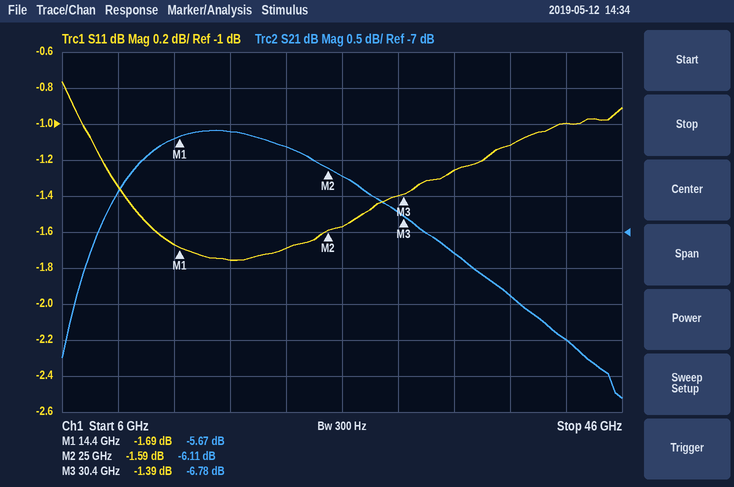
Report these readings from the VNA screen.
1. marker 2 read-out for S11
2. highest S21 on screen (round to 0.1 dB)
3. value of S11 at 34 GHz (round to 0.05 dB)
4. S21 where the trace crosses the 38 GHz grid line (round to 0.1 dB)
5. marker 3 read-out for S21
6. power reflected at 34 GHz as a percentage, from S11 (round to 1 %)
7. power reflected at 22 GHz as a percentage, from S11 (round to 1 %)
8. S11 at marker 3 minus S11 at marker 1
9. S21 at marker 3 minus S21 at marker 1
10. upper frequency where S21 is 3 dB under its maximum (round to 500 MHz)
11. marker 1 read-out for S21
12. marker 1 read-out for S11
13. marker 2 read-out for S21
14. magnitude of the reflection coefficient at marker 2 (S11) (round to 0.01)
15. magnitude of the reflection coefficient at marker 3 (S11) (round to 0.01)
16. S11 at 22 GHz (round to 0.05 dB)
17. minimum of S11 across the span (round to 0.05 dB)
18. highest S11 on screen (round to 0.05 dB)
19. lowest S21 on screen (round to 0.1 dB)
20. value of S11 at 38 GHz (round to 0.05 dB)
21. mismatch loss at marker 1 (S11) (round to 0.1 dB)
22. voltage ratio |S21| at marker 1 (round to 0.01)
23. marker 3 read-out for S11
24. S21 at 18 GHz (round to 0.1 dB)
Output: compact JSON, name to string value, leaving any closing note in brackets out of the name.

{"marker 2 read-out for S11": "-1.59 dB", "highest S21 on screen": "-5.6 dB", "value of S11 at 34 GHz": "-1.25 dB", "S21 where the trace crosses the 38 GHz grid line": "-7.9 dB", "marker 3 read-out for S21": "-6.78 dB", "power reflected at 34 GHz as a percentage, from S11": "75 %", "power reflected at 22 GHz as a percentage, from S11": "68 %", "S11 at marker 3 minus S11 at marker 1": "0.30 dB", "S21 at marker 3 minus S21 at marker 1": "-1.11 dB", "upper frequency where S21 is 3 dB under its maximum": "42.5 GHz", "marker 1 read-out for S21": "-5.67 dB", "marker 1 read-out for S11": "-1.69 dB", "marker 2 read-out for S21": "-6.11 dB", "magnitude of the reflection coefficient at marker 2 (S11)": "0.83", "magnitude of the reflection coefficient at marker 3 (S11)": "0.85", "S11 at 22 GHz": "-1.70 dB", "minimum of S11 across the span": "-1.75 dB", "highest S11 on screen": "-0.75 dB", "lowest S21 on screen": "-9.3 dB", "value of S11 at 38 GHz": "-1.10 dB", "mismatch loss at marker 1 (S11)": "4.9 dB", "voltage ratio |S21| at marker 1": "0.52", "marker 3 read-out for S11": "-1.39 dB", "S21 at 18 GHz": "-5.6 dB"}
